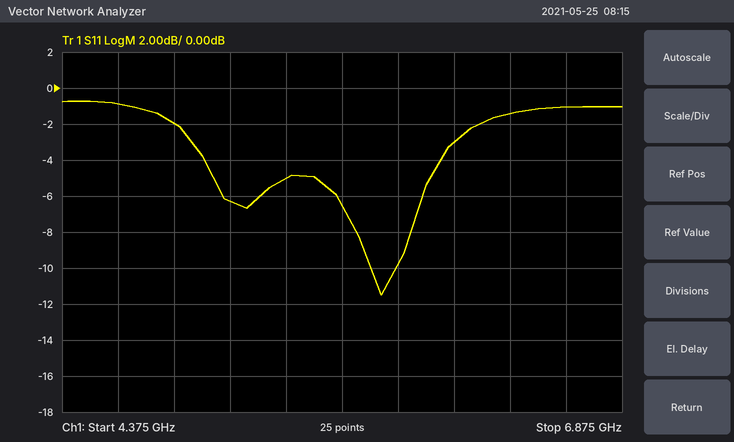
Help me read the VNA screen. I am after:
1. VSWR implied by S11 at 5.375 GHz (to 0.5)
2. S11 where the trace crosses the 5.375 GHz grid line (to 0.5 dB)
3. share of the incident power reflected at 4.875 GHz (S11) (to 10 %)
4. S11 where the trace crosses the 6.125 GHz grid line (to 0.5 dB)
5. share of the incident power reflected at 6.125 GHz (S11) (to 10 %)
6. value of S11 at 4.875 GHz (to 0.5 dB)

3.5
-5.0 dB
60 %
-3.0 dB
50 %
-2.0 dB
